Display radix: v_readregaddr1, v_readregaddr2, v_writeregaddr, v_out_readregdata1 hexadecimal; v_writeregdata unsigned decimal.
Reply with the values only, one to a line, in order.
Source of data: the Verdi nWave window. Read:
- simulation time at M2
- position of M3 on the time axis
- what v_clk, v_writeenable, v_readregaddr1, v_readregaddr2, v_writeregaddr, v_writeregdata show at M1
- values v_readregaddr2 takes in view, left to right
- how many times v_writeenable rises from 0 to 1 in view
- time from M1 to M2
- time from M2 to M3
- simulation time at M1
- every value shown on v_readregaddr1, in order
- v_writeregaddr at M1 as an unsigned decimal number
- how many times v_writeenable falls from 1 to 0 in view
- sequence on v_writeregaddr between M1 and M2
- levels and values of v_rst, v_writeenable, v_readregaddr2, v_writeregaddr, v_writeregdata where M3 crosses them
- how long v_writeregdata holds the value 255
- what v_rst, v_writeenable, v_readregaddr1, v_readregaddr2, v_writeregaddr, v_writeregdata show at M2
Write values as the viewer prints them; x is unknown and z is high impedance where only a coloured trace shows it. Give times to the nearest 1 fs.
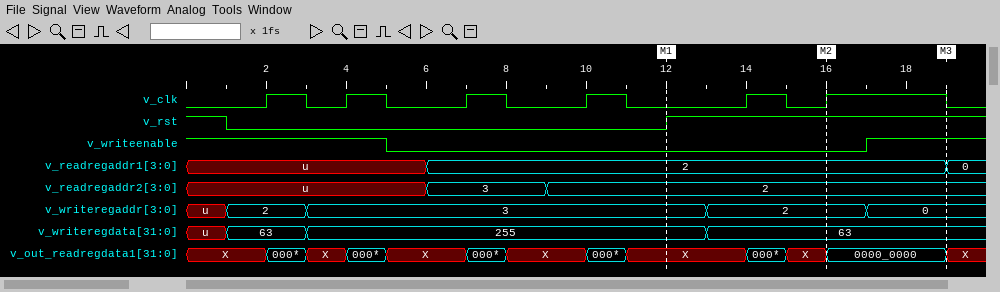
16 fs
19 fs
v_clk=0, v_writeenable=0, v_readregaddr1=2, v_readregaddr2=2, v_writeregaddr=3, v_writeregdata=255
u, 3, 2
1
4 fs
3 fs
12 fs
u, 2, 0
3
1
3, 2
v_rst=1, v_writeenable=1, v_readregaddr2=2, v_writeregaddr=0, v_writeregdata=63
10 fs
v_rst=1, v_writeenable=0, v_readregaddr1=2, v_readregaddr2=2, v_writeregaddr=2, v_writeregdata=63
